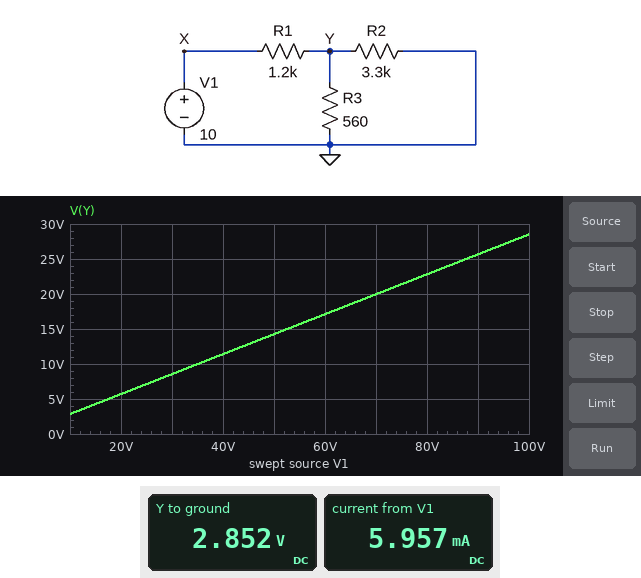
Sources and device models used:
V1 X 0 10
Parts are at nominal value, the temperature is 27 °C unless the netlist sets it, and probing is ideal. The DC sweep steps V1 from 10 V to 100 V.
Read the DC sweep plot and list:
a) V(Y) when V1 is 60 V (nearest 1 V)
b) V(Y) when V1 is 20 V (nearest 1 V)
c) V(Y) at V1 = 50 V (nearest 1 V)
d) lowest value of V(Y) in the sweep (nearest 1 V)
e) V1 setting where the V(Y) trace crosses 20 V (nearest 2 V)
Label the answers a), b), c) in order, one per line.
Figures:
a) 17 V
b) 6 V
c) 14 V
d) 3 V
e) 70 V
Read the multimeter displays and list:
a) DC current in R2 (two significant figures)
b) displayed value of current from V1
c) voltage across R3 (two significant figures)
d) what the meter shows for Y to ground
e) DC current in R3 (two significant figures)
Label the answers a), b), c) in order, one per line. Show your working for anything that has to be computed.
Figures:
a) (2.852 V) / 3.3 kΩ = 860 µA
b) 5.957 mA
c) 2.852 V = 2.9 V
d) 2.852 V
e) (2.852 V) / 560 Ω = 5.1 mA
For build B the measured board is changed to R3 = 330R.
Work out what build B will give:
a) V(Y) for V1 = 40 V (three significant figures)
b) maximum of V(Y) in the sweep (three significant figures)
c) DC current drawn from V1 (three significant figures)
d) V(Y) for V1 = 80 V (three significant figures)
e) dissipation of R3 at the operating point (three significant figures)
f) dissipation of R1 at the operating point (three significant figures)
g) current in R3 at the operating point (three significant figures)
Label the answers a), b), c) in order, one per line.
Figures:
a) 8.00 V
b) 20.0 V
c) 6.67 mA
d) 16.0 V
e) 12.1 mW
f) 53.3 mW
g) 6.06 mA
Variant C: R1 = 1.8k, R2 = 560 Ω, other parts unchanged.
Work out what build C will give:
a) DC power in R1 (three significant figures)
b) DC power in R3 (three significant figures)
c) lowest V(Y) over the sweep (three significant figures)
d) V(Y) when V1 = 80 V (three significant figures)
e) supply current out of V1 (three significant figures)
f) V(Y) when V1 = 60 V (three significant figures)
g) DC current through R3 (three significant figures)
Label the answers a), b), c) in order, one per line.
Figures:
a) 41.6 mW
b) 3.24 mW
c) 1.35 V
d) 10.8 V
e) 4.81 mA
f) 8.08 V
g) 2.40 mA
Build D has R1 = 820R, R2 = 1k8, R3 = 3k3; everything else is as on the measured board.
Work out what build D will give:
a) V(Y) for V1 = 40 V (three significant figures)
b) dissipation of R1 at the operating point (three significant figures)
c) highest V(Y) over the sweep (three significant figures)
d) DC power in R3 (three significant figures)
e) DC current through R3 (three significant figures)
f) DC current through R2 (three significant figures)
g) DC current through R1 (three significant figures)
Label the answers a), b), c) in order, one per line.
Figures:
a) 23.5 V
b) 20.8 mW
c) 58.7 V
d) 10.4 mW
e) 1.78 mA
f) 3.26 mA
g) 5.04 mA
